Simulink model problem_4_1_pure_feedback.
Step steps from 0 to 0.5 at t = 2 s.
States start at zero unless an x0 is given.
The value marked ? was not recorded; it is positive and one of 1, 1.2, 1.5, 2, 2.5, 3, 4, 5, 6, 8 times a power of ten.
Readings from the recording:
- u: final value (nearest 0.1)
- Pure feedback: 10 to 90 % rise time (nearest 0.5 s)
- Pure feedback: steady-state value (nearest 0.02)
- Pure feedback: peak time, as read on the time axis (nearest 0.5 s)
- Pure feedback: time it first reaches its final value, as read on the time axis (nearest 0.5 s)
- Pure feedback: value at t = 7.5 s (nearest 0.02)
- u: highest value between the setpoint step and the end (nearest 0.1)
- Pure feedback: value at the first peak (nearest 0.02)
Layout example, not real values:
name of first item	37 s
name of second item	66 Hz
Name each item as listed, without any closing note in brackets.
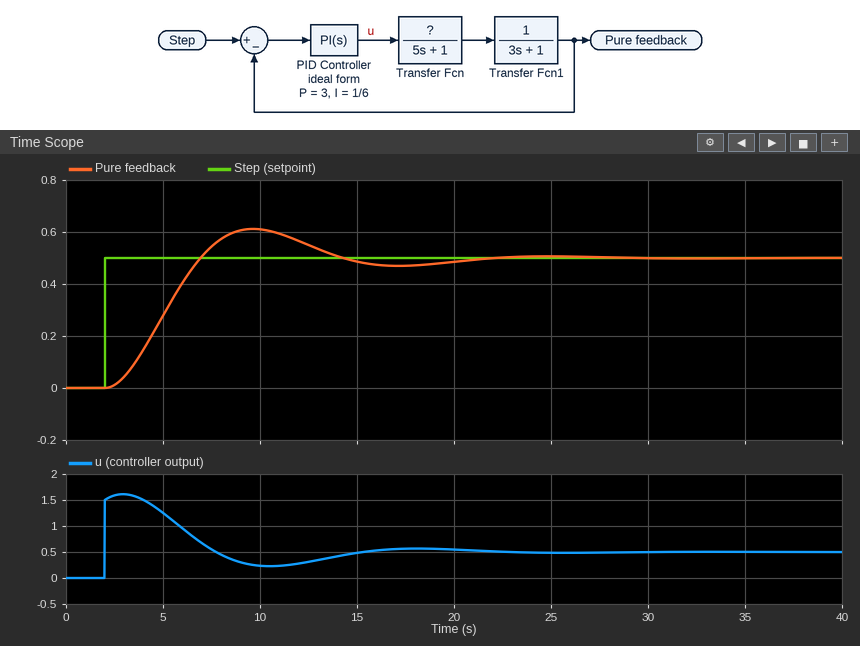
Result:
u: final value	0.5
Pure feedback: 10 to 90 % rise time	3.5 s
Pure feedback: steady-state value	0.50
Pure feedback: peak time, as read on the time axis	9.5 s
Pure feedback: time it first reaches its final value, as read on the time axis	7.0 s
Pure feedback: value at t = 7.5 s	0.54
u: highest value between the setpoint step and the end	1.6
Pure feedback: value at the first peak	0.62
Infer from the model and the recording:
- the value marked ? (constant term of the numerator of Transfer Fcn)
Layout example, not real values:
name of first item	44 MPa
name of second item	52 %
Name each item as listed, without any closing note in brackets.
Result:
the value marked ?	1
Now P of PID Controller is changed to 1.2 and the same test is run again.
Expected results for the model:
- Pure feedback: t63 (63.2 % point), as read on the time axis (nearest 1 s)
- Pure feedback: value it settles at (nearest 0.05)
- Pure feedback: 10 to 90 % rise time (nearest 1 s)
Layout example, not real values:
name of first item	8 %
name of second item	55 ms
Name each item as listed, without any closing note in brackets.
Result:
Pure feedback: t63 (63.2 % point), as read on the time axis	8 s
Pure feedback: value it settles at	0.50
Pure feedback: 10 to 90 % rise time	7 s
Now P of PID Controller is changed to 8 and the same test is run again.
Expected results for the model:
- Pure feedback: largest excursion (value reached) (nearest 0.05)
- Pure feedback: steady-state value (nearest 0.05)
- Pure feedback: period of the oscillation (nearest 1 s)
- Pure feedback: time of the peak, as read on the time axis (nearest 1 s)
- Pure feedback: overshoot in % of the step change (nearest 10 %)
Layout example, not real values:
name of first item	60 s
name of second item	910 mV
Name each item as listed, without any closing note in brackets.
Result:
Pure feedback: largest excursion (value reached)	0.70
Pure feedback: steady-state value	0.50
Pure feedback: period of the oscillation	9 s
Pure feedback: time of the peak, as read on the time axis	6 s
Pure feedback: overshoot in % of the step change	40 %
